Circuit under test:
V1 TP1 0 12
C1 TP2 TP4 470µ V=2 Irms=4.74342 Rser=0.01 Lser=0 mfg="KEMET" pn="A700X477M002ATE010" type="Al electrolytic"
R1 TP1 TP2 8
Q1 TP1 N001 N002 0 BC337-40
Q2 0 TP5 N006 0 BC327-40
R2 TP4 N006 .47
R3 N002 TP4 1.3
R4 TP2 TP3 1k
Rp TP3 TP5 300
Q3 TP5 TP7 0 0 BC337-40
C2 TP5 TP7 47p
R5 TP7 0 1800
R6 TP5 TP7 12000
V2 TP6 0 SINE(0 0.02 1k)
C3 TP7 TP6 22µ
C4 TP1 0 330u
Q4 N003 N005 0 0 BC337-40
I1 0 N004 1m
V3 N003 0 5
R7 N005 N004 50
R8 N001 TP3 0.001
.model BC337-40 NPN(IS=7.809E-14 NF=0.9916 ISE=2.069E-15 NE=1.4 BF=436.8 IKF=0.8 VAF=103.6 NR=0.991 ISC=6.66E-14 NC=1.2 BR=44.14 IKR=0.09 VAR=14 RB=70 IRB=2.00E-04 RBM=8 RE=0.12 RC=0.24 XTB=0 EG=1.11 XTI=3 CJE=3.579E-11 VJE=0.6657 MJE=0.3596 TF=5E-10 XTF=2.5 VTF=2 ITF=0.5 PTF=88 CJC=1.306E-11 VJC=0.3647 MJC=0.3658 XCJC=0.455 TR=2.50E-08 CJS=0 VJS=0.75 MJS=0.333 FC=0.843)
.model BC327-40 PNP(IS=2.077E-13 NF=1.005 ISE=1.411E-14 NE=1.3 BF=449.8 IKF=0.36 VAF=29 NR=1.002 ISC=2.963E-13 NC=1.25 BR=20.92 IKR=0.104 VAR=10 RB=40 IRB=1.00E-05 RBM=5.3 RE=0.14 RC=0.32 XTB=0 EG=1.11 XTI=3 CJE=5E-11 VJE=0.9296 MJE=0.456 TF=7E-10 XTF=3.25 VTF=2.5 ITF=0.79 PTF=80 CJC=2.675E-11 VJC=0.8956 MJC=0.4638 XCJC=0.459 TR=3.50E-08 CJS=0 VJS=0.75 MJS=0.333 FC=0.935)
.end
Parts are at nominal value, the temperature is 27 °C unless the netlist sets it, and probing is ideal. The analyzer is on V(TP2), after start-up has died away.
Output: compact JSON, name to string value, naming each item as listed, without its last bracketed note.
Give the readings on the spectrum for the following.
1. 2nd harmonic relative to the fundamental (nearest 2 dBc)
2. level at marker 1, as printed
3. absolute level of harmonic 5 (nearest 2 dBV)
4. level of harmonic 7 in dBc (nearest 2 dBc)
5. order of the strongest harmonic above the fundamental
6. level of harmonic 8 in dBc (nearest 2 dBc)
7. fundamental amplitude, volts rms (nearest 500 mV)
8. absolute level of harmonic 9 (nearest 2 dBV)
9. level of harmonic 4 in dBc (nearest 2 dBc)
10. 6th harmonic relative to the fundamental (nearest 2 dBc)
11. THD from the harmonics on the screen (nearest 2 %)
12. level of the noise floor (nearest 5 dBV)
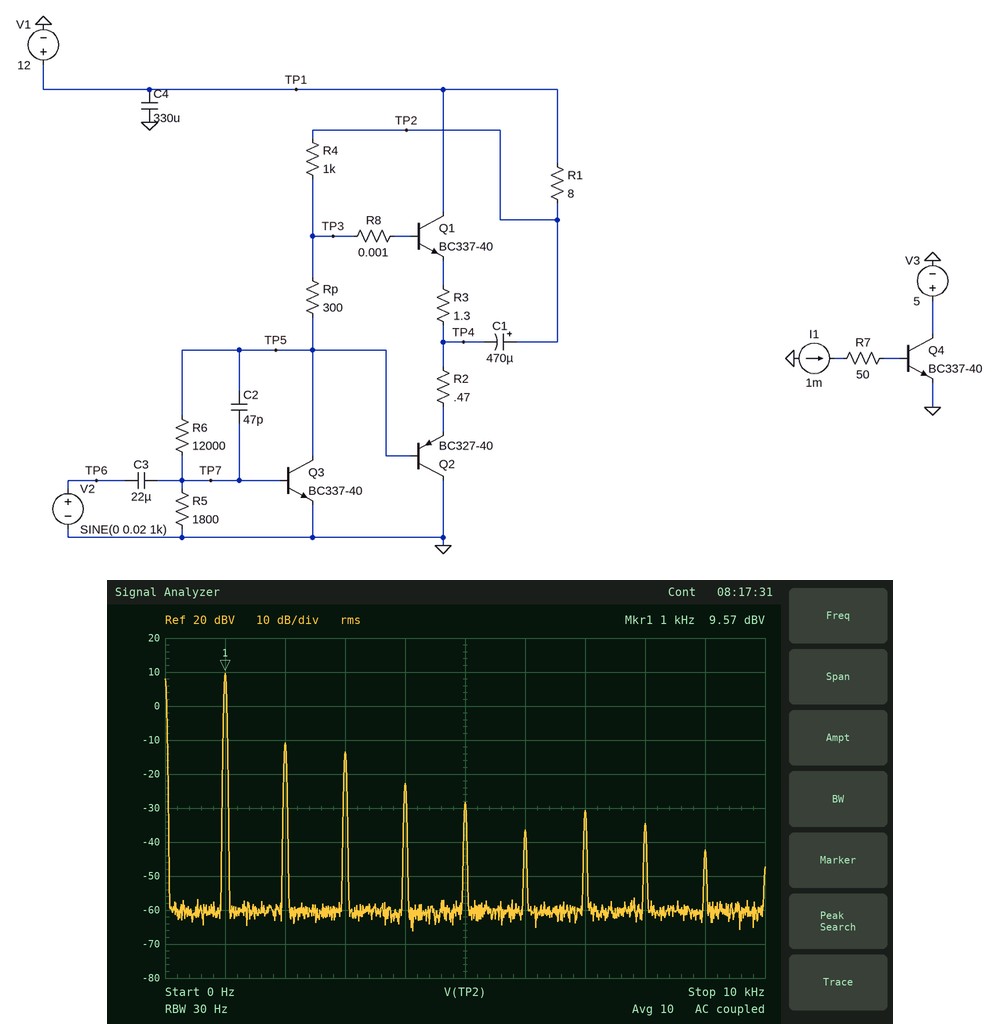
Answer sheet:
{"2nd harmonic relative to the fundamental": "-20 dBc", "level at marker 1, as printed": "9.57 dBV", "absolute level of harmonic 5": "-28 dBV", "level of harmonic 7 in dBc": "-40 dBc", "order of the strongest harmonic above the fundamental": "2", "level of harmonic 8 in dBc": "-44 dBc", "fundamental amplitude, volts rms": "3.0 V", "absolute level of harmonic 9": "-42 dBV", "level of harmonic 4 in dBc": "-32 dBc", "6th harmonic relative to the fundamental": "-46 dBc", "THD from the harmonics on the screen": "12 %", "level of the noise floor": "-60 dBV"}
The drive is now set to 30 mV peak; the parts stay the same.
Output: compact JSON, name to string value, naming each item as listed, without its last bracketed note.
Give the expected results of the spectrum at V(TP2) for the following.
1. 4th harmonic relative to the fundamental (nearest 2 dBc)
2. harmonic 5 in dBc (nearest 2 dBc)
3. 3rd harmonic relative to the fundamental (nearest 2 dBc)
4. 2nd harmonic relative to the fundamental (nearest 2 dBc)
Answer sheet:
{"4th harmonic relative to the fundamental": "-26 dBc", "harmonic 5 in dBc": "-34 dBc", "3rd harmonic relative to the fundamental": "-16 dBc", "2nd harmonic relative to the fundamental": "-28 dBc"}
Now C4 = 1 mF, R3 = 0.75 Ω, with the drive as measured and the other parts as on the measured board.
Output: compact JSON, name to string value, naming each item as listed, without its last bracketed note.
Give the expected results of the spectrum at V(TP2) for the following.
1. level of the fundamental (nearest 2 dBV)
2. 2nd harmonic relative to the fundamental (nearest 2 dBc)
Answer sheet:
{"level of the fundamental": "10 dBV", "2nd harmonic relative to the fundamental": "-22 dBc"}
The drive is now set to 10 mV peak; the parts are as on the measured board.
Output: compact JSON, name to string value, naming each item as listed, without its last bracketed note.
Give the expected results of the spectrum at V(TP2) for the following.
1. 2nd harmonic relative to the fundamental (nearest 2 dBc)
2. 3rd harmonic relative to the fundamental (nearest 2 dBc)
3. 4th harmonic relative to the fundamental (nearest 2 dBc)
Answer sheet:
{"2nd harmonic relative to the fundamental": "-24 dBc", "3rd harmonic relative to the fundamental": "-26 dBc", "4th harmonic relative to the fundamental": "-42 dBc"}
